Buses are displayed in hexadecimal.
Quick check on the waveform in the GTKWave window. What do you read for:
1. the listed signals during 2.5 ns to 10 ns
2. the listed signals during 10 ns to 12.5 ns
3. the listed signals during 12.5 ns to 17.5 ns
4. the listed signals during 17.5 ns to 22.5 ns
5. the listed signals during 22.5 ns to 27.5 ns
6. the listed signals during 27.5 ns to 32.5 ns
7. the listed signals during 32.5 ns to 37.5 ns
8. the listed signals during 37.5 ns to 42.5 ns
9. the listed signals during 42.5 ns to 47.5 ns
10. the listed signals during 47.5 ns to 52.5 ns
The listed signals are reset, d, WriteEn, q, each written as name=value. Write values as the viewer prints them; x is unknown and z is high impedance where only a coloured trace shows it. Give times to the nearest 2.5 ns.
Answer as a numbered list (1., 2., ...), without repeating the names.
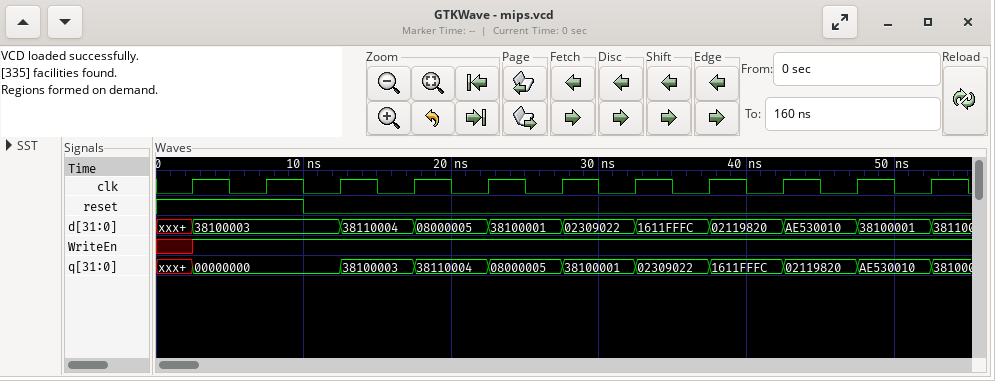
1. reset=1, d=38100003, WriteEn=1, q=00000000
2. reset=0, d=38100003, WriteEn=1, q=00000000
3. reset=0, d=38110004, WriteEn=1, q=38100003
4. reset=0, d=08000005, WriteEn=1, q=38110004
5. reset=0, d=38100001, WriteEn=1, q=08000005
6. reset=0, d=02309022, WriteEn=1, q=38100001
7. reset=0, d=1611FFFC, WriteEn=1, q=02309022
8. reset=0, d=02119820, WriteEn=1, q=1611FFFC
9. reset=0, d=AE530010, WriteEn=1, q=02119820
10. reset=0, d=38100001, WriteEn=1, q=AE530010
